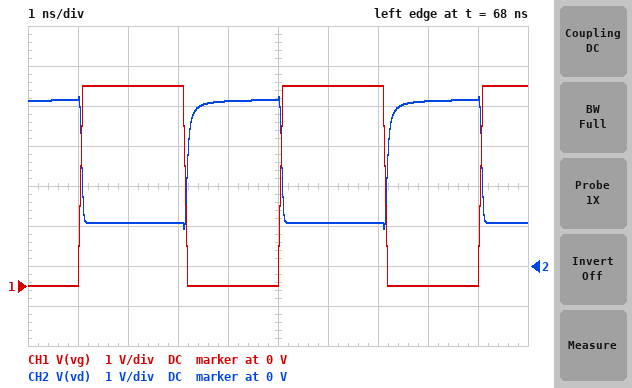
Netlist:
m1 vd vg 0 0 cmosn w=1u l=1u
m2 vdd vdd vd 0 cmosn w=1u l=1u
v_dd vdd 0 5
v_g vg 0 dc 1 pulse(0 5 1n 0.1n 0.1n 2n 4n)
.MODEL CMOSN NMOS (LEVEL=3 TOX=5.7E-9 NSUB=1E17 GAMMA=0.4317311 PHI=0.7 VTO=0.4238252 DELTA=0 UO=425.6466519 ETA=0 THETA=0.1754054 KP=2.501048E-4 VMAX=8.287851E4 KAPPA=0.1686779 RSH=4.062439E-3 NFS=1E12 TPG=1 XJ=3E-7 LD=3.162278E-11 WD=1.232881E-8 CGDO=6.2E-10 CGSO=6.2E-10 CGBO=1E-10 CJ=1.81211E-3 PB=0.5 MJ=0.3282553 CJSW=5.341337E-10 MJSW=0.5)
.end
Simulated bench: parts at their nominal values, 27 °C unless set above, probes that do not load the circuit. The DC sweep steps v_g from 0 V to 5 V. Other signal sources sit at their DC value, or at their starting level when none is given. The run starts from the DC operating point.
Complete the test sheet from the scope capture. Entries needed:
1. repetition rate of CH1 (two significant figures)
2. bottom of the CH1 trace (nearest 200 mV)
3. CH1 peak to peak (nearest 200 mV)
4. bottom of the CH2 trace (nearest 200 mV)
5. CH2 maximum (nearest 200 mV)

250 MHz
0 V
5.0 V
1.0 V
4.2 V
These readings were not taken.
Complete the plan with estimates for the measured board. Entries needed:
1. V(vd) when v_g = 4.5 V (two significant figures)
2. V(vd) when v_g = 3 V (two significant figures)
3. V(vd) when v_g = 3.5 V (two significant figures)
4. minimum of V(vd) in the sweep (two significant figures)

1.2 V
1.9 V
1.5 V
1.1 V
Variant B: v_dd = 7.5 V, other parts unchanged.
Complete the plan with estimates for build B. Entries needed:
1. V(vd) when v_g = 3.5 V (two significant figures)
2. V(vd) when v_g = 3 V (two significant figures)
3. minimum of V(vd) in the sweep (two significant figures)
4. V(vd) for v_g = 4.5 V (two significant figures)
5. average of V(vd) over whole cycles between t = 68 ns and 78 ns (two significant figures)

3.7 V
4.1 V
2.5 V
2.9 V
4.4 V
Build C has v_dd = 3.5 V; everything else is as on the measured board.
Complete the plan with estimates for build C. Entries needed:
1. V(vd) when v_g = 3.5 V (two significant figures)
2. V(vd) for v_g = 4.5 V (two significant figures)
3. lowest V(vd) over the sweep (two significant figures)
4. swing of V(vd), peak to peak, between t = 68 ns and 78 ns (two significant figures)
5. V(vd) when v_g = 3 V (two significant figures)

740 mV
610 mV
570 mV
2.5 V
840 mV
